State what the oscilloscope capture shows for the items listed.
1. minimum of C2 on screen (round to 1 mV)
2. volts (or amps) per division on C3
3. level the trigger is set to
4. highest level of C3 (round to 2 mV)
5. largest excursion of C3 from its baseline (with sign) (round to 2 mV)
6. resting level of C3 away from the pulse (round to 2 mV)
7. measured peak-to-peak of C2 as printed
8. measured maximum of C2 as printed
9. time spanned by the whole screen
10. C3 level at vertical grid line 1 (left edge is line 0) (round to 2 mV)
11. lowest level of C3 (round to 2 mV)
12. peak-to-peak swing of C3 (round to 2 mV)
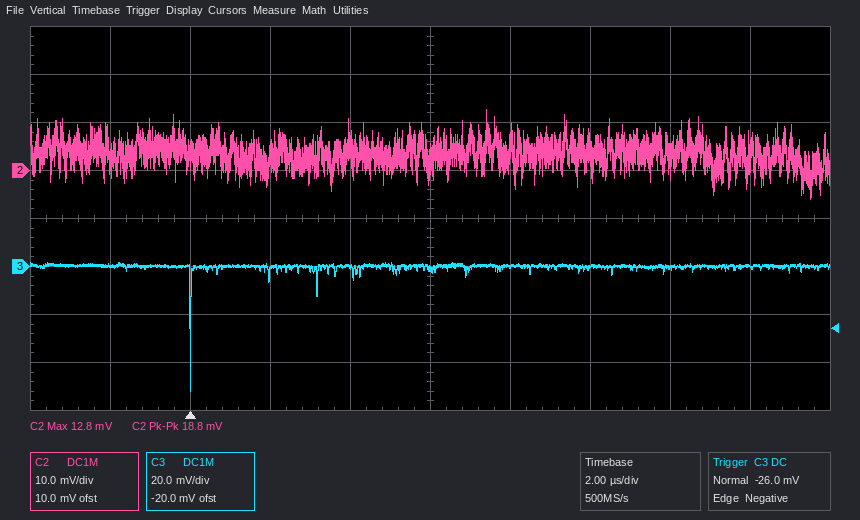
-6 mV
20 mV
-26.0 mV
2 mV
-52 mV
0 mV
18.8 mV
12.8 mV
20 µs
0 mV
-52 mV
54 mV
